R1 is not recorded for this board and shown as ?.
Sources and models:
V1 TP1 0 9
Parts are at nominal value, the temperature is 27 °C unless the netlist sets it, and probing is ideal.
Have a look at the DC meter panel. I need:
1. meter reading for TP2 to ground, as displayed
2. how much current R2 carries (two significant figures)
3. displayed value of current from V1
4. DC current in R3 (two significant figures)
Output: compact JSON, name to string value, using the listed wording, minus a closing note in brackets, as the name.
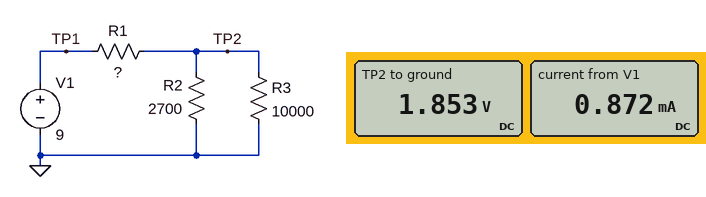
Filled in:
{"meter reading for TP2 to ground, as displayed": "1.853 V", "how much current R2 carries": "690 µA", "displayed value of current from V1": "0.872 mA", "DC current in R3": "190 µA"}
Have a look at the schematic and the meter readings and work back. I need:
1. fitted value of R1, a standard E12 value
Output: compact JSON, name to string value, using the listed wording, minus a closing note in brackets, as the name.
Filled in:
{"fitted value of R1, a standard E12 value": "8.2 kΩ"}
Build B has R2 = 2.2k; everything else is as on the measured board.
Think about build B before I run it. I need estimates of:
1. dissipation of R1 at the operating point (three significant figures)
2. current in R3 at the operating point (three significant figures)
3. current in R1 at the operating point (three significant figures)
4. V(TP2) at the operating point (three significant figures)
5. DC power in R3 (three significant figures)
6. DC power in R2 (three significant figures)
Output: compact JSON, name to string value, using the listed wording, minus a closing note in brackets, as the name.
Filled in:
{"dissipation of R1 at the operating point": "6.64 mW", "current in R3 at the operating point": "162 µA", "current in R1 at the operating point": "900 µA", "V(TP2) at the operating point": "1.62 V", "DC power in R3": "263 µW", "DC power in R2": "1.20 mW"}
